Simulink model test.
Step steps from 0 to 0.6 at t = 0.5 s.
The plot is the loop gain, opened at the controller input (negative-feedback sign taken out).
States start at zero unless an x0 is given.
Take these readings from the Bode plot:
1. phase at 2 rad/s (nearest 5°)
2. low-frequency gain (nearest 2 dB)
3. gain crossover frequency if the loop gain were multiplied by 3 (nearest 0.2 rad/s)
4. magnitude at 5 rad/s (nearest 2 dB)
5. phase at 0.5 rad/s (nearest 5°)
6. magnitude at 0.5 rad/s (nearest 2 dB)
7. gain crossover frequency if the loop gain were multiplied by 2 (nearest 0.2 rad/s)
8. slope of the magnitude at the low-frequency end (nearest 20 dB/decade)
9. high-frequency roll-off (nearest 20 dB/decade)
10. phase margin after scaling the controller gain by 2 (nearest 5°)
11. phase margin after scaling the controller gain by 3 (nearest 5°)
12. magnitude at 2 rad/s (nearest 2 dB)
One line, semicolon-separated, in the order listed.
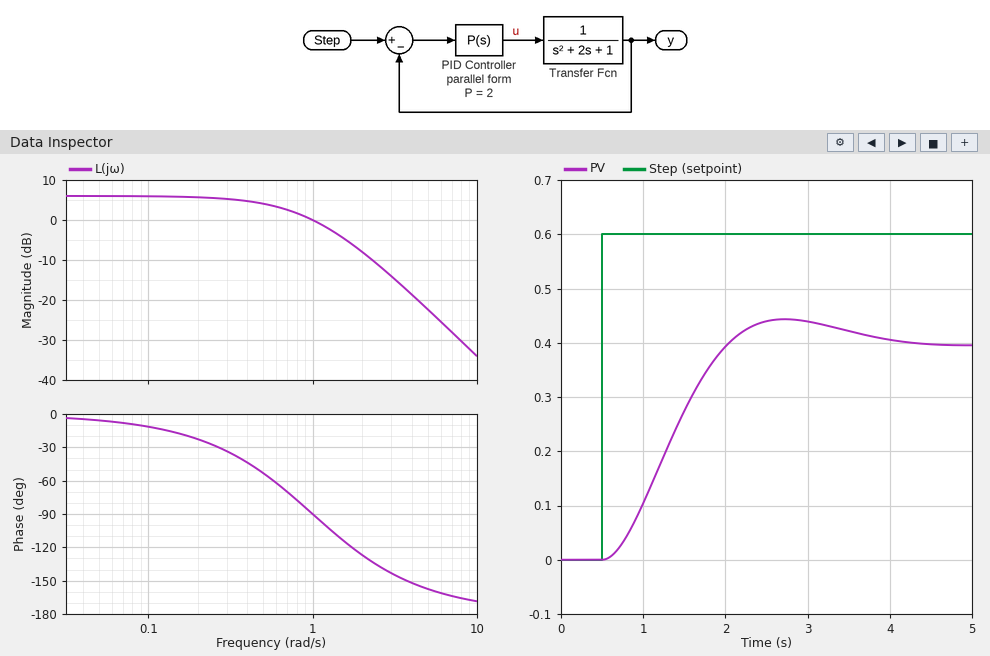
-125°; 6 dB; 2.2 rad/s; -22 dB; -55°; 4 dB; 1.8 rad/s; 0 dB/decade; -40 dB/decade; 60°; 50°; -8 dB
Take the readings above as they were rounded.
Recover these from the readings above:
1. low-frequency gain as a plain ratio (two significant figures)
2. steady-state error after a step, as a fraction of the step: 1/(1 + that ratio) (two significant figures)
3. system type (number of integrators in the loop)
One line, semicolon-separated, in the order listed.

2.0; 0.33; 0
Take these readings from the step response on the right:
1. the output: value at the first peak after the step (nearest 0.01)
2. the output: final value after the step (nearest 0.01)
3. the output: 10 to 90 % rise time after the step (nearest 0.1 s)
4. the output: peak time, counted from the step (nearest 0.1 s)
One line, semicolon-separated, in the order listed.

0.44; 0.40; 1.0 s; 2.2 s
